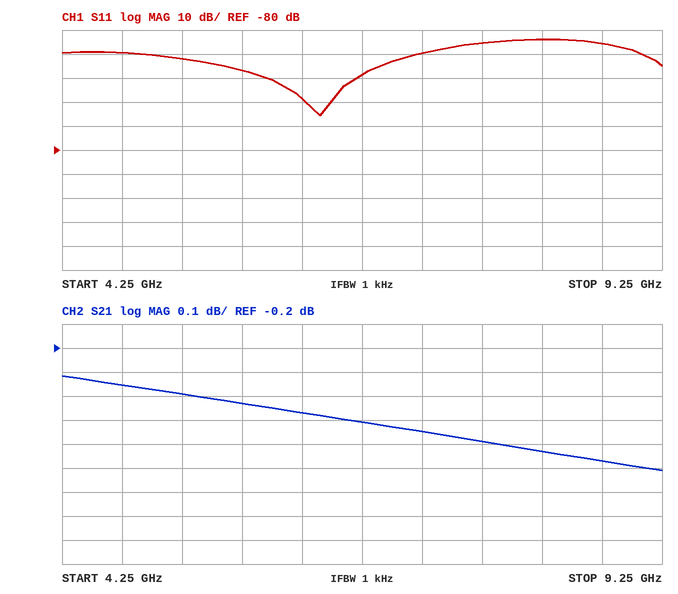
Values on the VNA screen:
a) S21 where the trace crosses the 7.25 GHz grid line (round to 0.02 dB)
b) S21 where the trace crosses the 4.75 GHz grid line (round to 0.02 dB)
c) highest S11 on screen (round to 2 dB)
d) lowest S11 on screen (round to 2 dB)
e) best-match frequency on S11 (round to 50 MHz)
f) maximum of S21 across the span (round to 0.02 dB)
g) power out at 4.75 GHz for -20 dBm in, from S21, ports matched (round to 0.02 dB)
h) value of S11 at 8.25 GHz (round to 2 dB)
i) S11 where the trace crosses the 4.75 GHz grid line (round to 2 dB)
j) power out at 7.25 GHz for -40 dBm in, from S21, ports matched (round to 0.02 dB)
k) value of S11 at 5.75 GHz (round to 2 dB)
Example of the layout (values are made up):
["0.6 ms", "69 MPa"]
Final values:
["-0.54 dB", "-0.36 dB", "-34 dB", "-66 dB", "6.40 GHz", "-0.32 dB", "-20.36 dBm", "-34 dB", "-40 dB", "-40.54 dBm", "-46 dB"]
